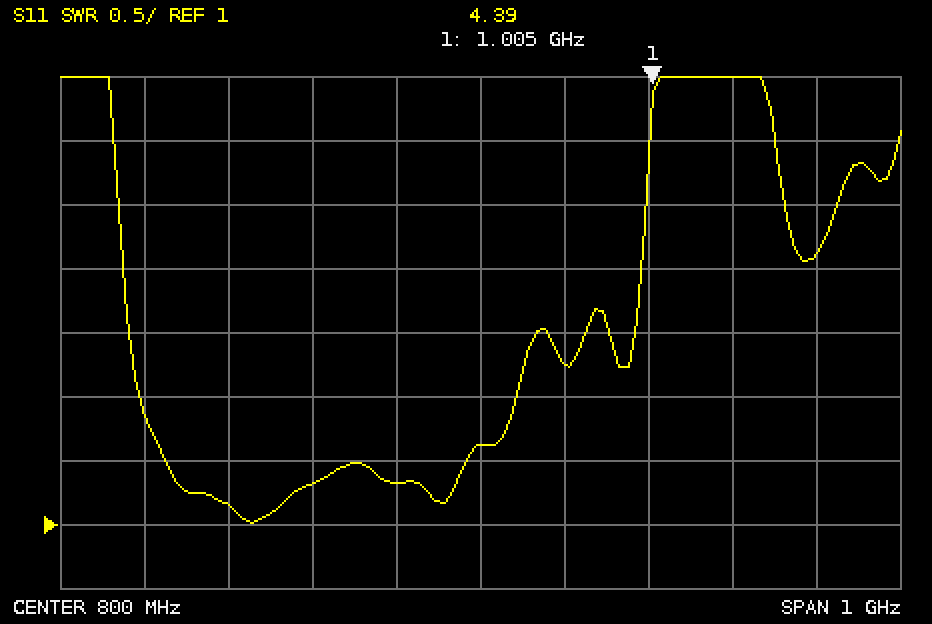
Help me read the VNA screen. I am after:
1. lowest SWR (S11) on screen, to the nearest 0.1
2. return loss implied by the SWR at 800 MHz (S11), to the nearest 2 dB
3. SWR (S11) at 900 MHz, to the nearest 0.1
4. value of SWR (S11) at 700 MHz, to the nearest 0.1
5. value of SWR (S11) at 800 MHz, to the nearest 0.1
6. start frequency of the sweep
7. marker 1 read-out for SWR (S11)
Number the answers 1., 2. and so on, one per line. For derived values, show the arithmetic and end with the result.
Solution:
1. 1.0
2. −20 log10((1.6 − 1)/(1.6 + 1)) ≈ 12.7 dB, so 12 dB to the nearest 2 dB
3. 2.3
4. 1.3
5. 1.6
6. 300 MHz
7. 4.39
